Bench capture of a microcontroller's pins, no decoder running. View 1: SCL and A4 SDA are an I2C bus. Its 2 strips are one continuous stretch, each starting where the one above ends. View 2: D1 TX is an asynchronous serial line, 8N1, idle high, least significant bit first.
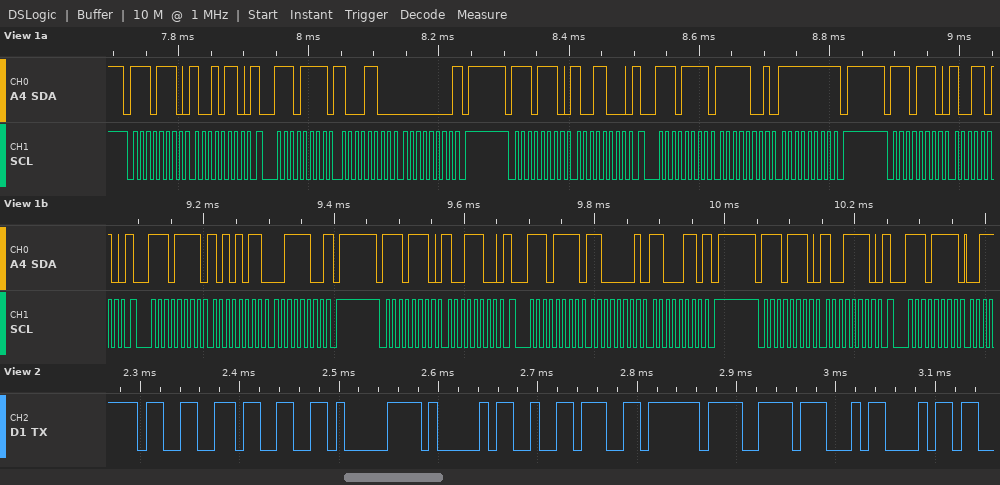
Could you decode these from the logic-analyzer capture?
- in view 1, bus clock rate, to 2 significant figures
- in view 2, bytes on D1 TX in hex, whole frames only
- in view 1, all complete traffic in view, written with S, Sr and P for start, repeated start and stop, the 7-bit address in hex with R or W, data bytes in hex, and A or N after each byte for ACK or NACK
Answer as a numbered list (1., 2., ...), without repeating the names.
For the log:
1. 100 kHz
2. 0x33 0x33 0xC1 0x41 0xB2 0xF6 0xCF 0x47 0x68
3. S 77W A 96 A Sr 77R A 8C A 00 N P S 77W A 98 A Sr 77R A F9 A FF N P S 77W A 9A A Sr 77R A AB A 3C N P S 77W A 9C A Sr 77R A C1 A C6 N P S 77W A 9E A Sr 77R A
